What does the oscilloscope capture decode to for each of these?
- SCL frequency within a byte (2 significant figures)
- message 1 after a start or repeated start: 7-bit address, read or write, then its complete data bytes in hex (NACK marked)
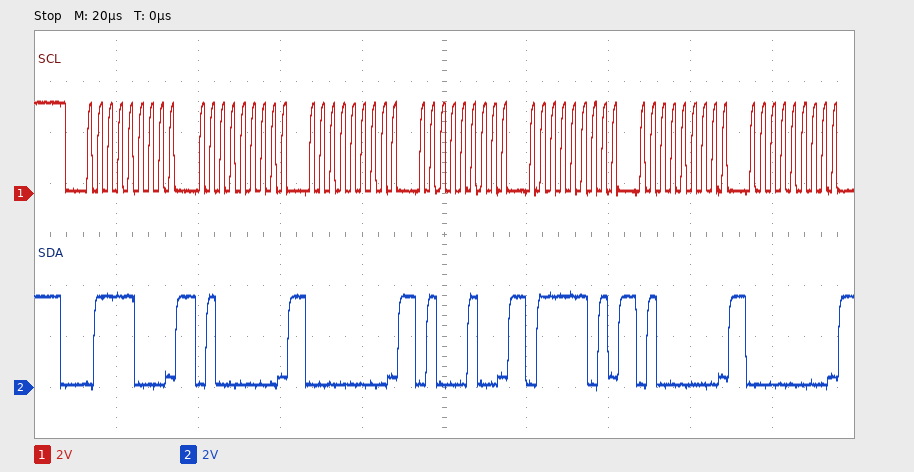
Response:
400 kHz
0x3C write: 40 00 44 7D 40 00
